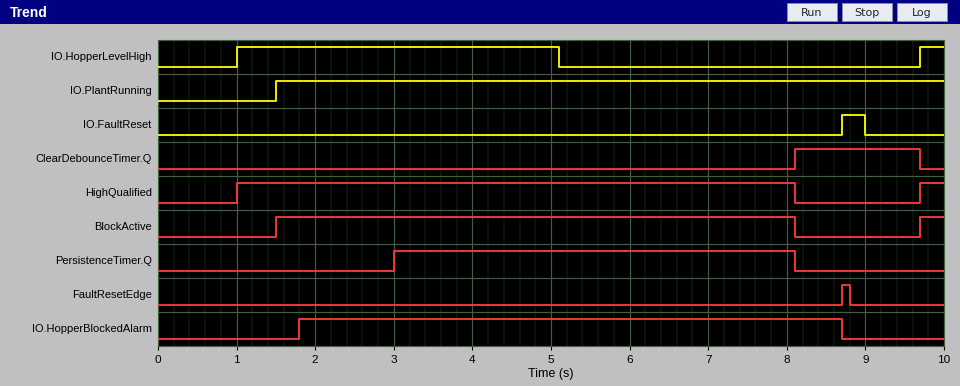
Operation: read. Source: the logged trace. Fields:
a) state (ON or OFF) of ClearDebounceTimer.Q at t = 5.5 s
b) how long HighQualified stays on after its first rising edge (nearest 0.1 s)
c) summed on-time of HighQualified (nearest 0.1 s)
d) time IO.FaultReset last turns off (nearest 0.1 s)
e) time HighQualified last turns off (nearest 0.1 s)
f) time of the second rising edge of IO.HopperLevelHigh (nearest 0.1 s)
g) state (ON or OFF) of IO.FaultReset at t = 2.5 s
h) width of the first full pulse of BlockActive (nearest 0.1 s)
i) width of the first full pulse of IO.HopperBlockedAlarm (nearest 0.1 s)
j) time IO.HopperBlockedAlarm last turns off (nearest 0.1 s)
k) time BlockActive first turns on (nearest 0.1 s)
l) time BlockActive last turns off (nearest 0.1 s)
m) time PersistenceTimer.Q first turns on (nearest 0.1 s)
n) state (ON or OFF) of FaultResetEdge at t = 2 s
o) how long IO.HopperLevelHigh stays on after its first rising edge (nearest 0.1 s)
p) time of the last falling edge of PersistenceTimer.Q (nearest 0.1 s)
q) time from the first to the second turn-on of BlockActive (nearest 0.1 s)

OFF
7.1 s
7.4 s
9.0 s
8.1 s
9.7 s
OFF
6.6 s
6.9 s
8.7 s
1.5 s
8.1 s
3.0 s
OFF
4.1 s
8.1 s
8.2 s
